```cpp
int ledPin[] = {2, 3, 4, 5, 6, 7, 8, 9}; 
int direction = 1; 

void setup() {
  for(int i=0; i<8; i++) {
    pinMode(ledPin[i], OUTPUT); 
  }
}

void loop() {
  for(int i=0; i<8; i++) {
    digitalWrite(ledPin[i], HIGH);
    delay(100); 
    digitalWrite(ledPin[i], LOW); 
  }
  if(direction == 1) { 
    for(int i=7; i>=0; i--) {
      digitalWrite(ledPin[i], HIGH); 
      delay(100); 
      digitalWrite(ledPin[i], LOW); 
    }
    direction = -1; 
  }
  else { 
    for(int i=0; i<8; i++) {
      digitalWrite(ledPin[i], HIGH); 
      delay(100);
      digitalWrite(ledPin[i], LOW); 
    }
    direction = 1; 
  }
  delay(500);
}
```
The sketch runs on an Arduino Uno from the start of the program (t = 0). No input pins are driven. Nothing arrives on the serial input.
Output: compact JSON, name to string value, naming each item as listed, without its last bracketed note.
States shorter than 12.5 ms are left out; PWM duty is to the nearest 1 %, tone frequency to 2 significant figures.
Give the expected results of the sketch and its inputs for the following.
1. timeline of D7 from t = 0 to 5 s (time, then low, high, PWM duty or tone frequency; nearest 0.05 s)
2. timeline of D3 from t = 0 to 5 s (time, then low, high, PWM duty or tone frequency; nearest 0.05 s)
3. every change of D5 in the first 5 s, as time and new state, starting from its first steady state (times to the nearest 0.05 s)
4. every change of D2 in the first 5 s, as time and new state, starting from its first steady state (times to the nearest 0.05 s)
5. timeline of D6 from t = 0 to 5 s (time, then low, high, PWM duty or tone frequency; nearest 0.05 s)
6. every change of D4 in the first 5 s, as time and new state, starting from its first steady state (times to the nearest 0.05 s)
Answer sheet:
{"timeline of D7 from t = 0 to 5 s": "0 s low; 0.5 s high; 0.6 s low; 1 s high; 1.1 s low; 2.6 s high; 2.7 s low; 3.4 s high; 3.5 s low; 4.7 s high; 4.8 s low", "timeline of D3 from t = 0 to 5 s": "0 s low; 0.1 s high; 0.2 s low; 1.4 s high; 1.5 s low; 2.2 s high; 2.3 s low; 3 s high; 3.1 s low; 4.3 s high; 4.4 s low", "every change of D5 in the first 5 s, as time and new state, starting from its first steady state": "0 s low; 0.3 s high; 0.4 s low; 1.2 s high; 1.3 s low; 2.4 s high; 2.5 s low; 3.2 s high; 3.3 s low; 4.5 s high; 4.6 s low", "every change of D2 in the first 5 s, as time and new state, starting from its first steady state": "0 s high; 0.1 s low; 1.5 s high; 1.6 s low; 2.1 s high; 2.2 s low; 2.9 s high; 3 s low; 4.2 s high; 4.3 s low", "timeline of D6 from t = 0 to 5 s": "0 s low; 0.4 s high; 0.5 s low; 1.1 s high; 1.2 s low; 2.5 s high; 2.6 s low; 3.3 s high; 3.4 s low; 4.6 s high; 4.7 s low", "every change of D4 in the first 5 s, as time and new state, starting from its first steady state": "0 s low; 0.2 s high; 0.3 s low; 1.3 s high; 1.4 s low; 2.3 s high; 2.4 s low; 3.1 s high; 3.2 s low; 4.4 s high; 4.5 s low"}
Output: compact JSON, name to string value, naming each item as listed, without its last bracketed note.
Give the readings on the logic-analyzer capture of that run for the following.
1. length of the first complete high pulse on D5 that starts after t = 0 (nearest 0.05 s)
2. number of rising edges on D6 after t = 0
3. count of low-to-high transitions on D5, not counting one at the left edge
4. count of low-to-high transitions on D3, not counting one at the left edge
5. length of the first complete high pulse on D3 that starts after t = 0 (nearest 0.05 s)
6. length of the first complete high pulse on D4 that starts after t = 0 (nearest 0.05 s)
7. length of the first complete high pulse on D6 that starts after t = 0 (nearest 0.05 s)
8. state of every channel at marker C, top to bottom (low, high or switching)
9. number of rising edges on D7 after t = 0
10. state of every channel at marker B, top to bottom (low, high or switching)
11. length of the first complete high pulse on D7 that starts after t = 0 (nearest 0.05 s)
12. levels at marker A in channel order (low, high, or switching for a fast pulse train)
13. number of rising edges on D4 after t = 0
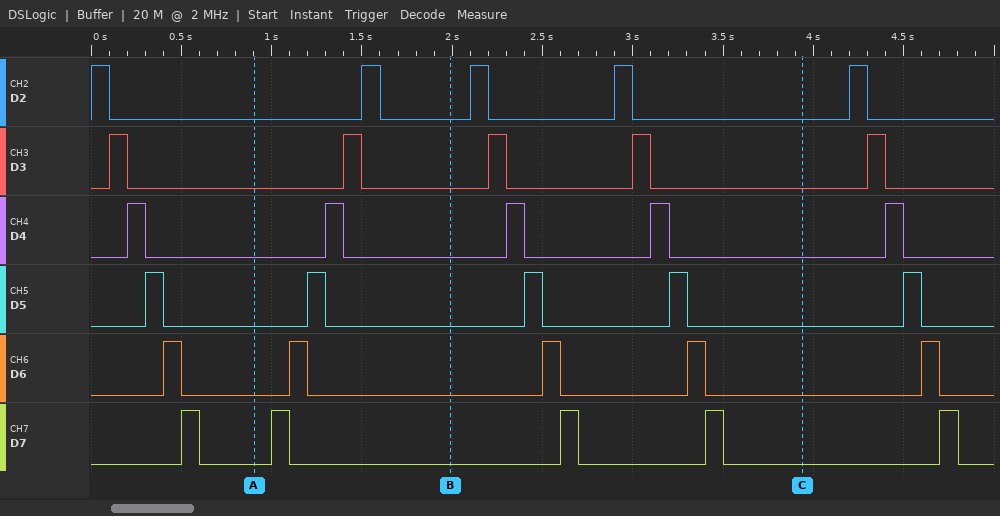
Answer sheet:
{"length of the first complete high pulse on D5 that starts after t = 0": "0.10 s", "number of rising edges on D6 after t = 0": "5", "count of low-to-high transitions on D5, not counting one at the left edge": "5", "count of low-to-high transitions on D3, not counting one at the left edge": "5", "length of the first complete high pulse on D3 that starts after t = 0": "0.10 s", "length of the first complete high pulse on D4 that starts after t = 0": "0.10 s", "length of the first complete high pulse on D6 that starts after t = 0": "0.10 s", "state of every channel at marker C, top to bottom": "D2 low, D3 low, D4 low, D5 low, D6 low, D7 low", "number of rising edges on D7 after t = 0": "5", "state of every channel at marker B, top to bottom": "D2 low, D3 low, D4 low, D5 low, D6 low, D7 low", "length of the first complete high pulse on D7 that starts after t = 0": "0.10 s", "levels at marker A in channel order": "D2 low, D3 low, D4 low, D5 low, D6 low, D7 low", "number of rising edges on D4 after t = 0": "5"}
